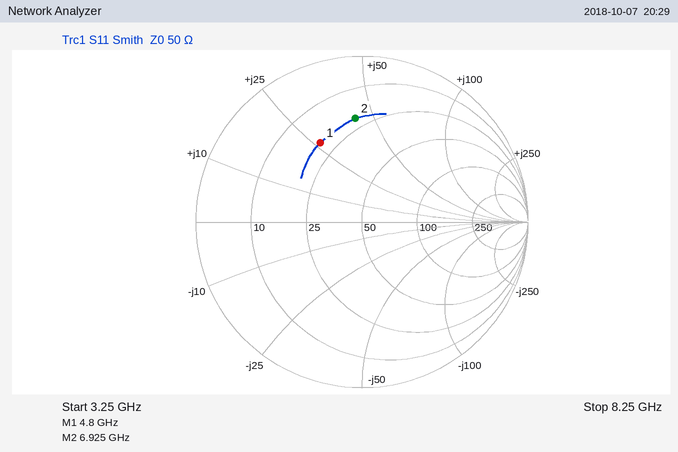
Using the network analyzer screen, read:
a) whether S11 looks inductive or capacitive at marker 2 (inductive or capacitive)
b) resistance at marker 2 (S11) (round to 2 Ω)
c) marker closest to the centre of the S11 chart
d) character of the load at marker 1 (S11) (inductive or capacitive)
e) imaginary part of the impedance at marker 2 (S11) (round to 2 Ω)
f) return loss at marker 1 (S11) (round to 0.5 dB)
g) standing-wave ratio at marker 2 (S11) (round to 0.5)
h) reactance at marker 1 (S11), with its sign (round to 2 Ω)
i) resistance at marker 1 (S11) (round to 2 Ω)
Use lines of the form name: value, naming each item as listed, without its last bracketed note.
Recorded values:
whether S11 looks inductive or capacitive at marker 2: inductive
resistance at marker 2 (S11): 20 Ω
marker closest to the centre of the S11 chart: marker 1
character of the load at marker 1 (S11): inductive
imaginary part of the impedance at marker 2 (S11): +42 Ω
return loss at marker 1 (S11): 5.5 dB
standing-wave ratio at marker 2 (S11): 4.5
reactance at marker 1 (S11), with its sign: +26 Ω
resistance at marker 1 (S11): 20 Ω
